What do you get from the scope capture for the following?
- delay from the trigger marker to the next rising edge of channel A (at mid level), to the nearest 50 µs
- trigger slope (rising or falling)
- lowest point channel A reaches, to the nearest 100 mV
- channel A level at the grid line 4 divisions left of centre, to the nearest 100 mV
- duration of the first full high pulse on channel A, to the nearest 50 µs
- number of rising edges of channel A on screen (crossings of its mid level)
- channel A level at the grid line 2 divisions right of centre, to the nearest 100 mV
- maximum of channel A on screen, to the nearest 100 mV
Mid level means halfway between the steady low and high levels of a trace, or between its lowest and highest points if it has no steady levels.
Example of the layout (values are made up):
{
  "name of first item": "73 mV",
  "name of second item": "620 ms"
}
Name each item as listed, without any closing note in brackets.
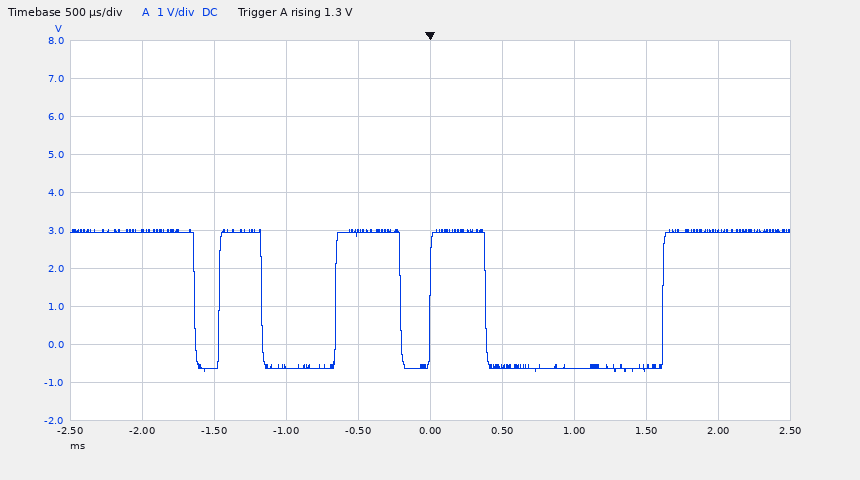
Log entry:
{
  "delay from the trigger marker to the next rising edge of channel A (at mid level), to the nearest 50 µs": "1.60 ms",
  "trigger slope": "rising",
  "lowest point channel A reaches, to the nearest 100 mV": "-700 mV",
  "channel A level at the grid line 4 divisions left of centre, to the nearest 100 mV": "3.0 V",
  "duration of the first full high pulse on channel A, to the nearest 50 µs": "300 µs",
  "number of rising edges of channel A on screen": "4",
  "channel A level at the grid line 2 divisions right of centre, to the nearest 100 mV": "-600 mV",
  "maximum of channel A on screen, to the nearest 100 mV": "3.0 V"
}
